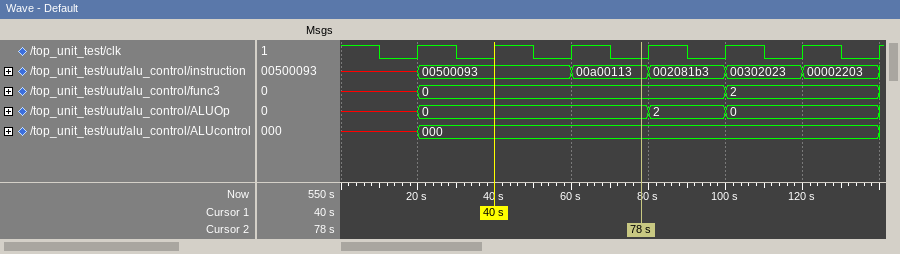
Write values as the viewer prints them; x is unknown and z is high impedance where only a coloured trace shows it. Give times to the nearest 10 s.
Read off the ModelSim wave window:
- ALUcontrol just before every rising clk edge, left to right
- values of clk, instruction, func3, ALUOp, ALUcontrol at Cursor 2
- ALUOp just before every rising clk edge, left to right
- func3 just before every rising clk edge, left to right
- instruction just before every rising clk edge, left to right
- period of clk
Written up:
x, 000, 000, 000, 000, 000, 000
clk=0, instruction=00a00113, func3=0, ALUOp=0, ALUcontrol=000
x, 0, 0, 0, 2, 0, 0
x, 0, 0, 0, 0, 2, 2
x, 00500093, 00500093, 00a00113, 002081b3, 00302023, 00002203
20 s
